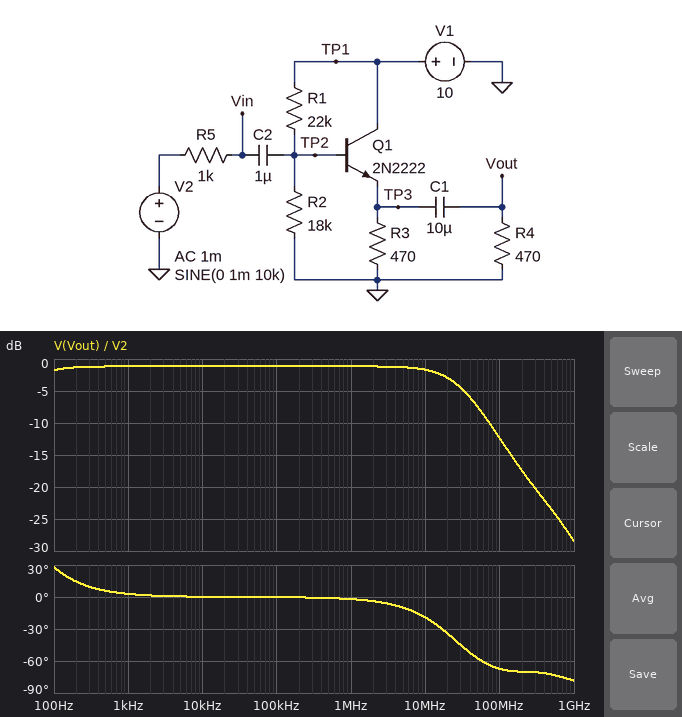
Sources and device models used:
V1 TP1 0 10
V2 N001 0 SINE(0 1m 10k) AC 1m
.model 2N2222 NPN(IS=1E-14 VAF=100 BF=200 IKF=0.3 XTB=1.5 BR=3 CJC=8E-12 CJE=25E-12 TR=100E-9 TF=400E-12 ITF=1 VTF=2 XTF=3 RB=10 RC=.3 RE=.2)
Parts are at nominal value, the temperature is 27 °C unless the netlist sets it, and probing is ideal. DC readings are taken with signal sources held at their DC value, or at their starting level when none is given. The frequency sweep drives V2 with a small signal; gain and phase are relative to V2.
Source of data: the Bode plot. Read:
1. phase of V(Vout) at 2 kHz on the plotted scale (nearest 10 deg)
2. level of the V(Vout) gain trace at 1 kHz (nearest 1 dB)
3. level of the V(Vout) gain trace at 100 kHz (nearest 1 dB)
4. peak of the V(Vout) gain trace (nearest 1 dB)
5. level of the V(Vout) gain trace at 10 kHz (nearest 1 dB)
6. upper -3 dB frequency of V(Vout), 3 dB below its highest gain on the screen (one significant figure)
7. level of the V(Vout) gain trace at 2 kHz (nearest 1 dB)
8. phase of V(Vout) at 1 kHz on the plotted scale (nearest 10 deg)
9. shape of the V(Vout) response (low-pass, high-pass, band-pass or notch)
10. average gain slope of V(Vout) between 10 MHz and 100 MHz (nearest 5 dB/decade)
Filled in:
0 deg
-1 dB
-1 dB
-1 dB
-1 dB
30 MHz
-1 dB
0 deg
low-pass
-10 dB/decade
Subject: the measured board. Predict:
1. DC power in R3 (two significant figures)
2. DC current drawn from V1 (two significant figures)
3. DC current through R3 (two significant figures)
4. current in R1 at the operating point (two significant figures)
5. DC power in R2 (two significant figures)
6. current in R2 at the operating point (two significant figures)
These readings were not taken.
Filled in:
25 mW
7.6 mA
7.3 mA
270 µA
960 µW
230 µA
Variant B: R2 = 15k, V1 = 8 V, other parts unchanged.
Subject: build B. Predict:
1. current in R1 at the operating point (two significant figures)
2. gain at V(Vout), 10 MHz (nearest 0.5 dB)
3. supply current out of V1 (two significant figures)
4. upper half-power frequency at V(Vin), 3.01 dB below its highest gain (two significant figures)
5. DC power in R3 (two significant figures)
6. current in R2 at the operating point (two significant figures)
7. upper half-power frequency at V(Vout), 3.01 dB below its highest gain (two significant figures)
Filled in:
230 µA
-2.0 dB
5.2 mA
19 MHz
12 mW
200 µA
26 MHz
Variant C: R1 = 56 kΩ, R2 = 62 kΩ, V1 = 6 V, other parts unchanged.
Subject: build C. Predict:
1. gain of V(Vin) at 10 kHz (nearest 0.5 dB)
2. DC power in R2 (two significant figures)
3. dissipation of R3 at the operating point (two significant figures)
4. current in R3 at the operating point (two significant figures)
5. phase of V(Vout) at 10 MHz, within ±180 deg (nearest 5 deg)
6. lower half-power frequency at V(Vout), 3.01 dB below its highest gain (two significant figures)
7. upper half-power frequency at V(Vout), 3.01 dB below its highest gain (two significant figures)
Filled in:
-0.5 dB
110 µW
7.6 mW
4.0 mA
-25 deg
36 Hz
22 MHz
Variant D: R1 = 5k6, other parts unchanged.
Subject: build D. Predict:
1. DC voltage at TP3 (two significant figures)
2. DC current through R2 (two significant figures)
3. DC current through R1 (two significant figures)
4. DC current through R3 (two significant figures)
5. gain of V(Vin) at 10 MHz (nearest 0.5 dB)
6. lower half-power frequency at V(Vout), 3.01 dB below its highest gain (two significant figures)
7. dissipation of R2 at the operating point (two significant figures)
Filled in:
6.6 V
410 µA
480 µA
14 mA
-2.5 dB
52 Hz
3.0 mW
